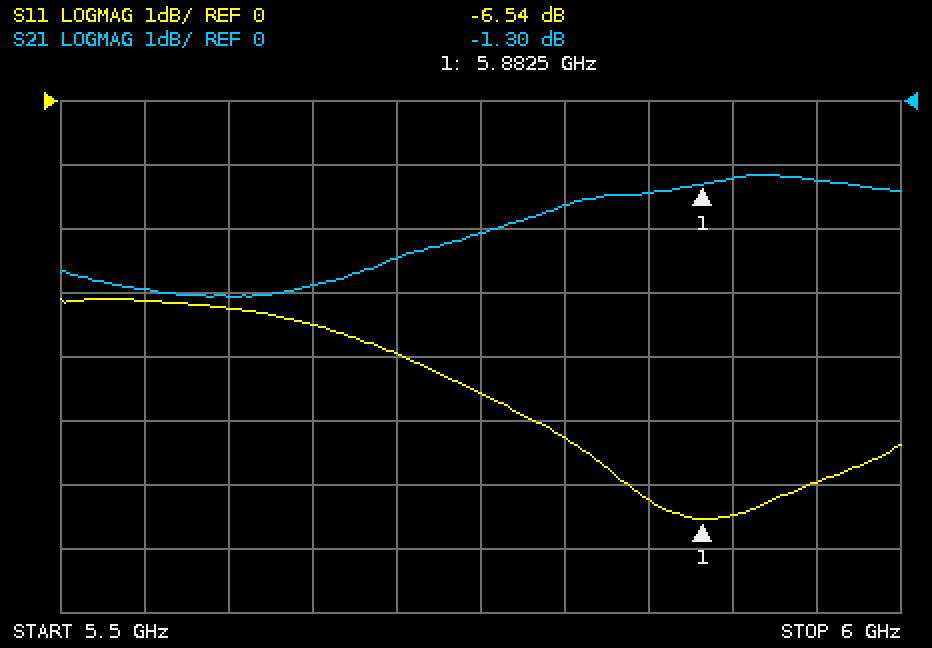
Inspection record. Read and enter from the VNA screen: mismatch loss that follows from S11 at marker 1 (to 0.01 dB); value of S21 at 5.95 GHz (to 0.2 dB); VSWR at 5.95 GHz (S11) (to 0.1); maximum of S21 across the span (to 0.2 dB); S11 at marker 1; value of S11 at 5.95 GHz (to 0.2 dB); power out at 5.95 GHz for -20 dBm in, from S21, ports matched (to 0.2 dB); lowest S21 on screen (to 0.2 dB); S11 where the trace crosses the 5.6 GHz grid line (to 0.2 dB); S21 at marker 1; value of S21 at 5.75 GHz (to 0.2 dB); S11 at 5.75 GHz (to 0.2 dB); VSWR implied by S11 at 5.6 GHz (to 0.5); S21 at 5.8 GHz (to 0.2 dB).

1.09 dB
-1.2 dB
3.0
-1.2 dB
-6.54 dB
-6.0 dB
-21.2 dBm
-3.0 dB
-3.2 dB
-1.30 dB
-2.0 dB
-4.6 dB
5.5
-1.6 dB
